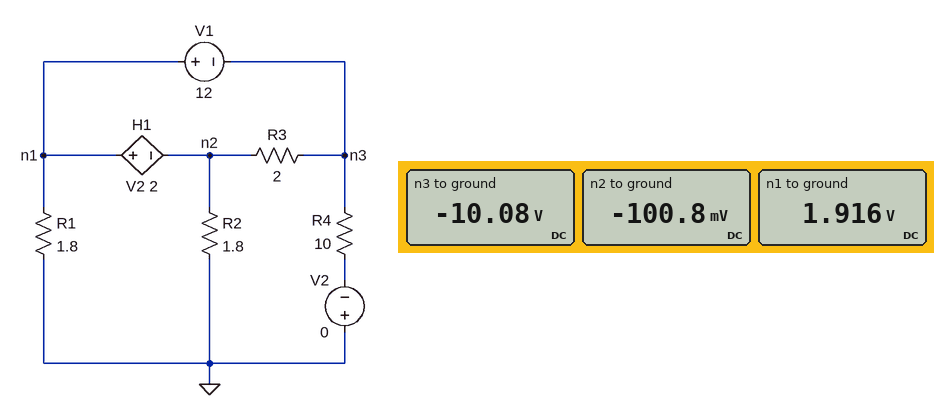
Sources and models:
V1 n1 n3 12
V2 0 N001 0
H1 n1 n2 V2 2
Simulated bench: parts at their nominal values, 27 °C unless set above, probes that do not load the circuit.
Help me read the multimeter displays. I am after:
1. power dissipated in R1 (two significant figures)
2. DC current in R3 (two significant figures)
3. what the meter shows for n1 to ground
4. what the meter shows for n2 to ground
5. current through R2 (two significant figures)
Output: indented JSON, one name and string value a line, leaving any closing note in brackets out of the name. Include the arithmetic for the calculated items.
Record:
{
  "power dissipated in R1": "(1.916 V)^2 / 1.8 Ω = 2.0 W",
  "DC current in R3": "(-100.8 mV - (-10.08 V)) / 2 Ω = 5.0 A",
  "what the meter shows for n1 to ground": "1.916 V",
  "what the meter shows for n2 to ground": "-100.8 mV",
  "current through R2": "(0 V - (-100.8 mV)) / 1.8 Ω = 56 mA"
}
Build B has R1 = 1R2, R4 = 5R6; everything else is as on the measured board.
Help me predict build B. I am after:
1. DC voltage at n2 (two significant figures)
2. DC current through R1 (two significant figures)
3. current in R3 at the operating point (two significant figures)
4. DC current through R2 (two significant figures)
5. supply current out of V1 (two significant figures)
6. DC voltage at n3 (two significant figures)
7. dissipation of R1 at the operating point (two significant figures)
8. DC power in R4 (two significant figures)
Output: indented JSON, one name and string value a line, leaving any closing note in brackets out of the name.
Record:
{
  "DC voltage at n2": "-810 mV",
  "DC current through R1": "2.1 A",
  "current in R3 at the operating point": "4.3 A",
  "DC current through R2": "450 mA",
  "supply current out of V1": "6.0 A",
  "DC voltage at n3": "-9.4 V",
  "dissipation of R1 at the operating point": "5.5 W",
  "DC power in R4": "16 W"
}
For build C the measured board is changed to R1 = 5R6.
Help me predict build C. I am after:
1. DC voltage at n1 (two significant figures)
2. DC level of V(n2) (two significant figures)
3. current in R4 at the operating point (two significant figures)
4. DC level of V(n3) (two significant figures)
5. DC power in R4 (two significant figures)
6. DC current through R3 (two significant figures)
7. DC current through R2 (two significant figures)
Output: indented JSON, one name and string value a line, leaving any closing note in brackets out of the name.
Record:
{
  "DC voltage at n1": "2.7 V",
  "DC level of V(n2)": "820 mV",
  "current in R4 at the operating point": "930 mA",
  "DC level of V(n3)": "-9.3 V",
  "DC power in R4": "8.7 W",
  "DC current through R3": "5.1 A",
  "DC current through R2": "450 mA"
}
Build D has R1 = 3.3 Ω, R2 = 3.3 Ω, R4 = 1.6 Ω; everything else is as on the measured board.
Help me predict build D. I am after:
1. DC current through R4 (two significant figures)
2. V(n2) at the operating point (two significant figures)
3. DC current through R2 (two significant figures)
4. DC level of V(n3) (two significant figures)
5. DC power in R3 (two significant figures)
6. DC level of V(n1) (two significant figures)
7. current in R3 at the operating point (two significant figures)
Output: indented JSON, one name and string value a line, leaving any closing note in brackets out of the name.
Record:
{
  "DC current through R4": "2.8 A",
  "V(n2) at the operating point": "1.8 V",
  "DC current through R2": "560 mA",
  "DC level of V(n3)": "-4.5 V",
  "DC power in R3": "20 W",
  "DC level of V(n1)": "7.5 V",
  "current in R3 at the operating point": "3.2 A"
}
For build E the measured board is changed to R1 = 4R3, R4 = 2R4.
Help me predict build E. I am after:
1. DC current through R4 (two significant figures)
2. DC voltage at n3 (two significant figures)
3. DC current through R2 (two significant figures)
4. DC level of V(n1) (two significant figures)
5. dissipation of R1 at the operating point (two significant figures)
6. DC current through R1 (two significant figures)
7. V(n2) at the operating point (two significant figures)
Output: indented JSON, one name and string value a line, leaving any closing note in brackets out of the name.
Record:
{
  "DC current through R4": "2.4 A",
  "DC voltage at n3": "-5.7 V",
  "DC current through R2": "890 mA",
  "DC level of V(n1)": "6.3 V",
  "dissipation of R1 at the operating point": "9.3 W",
  "DC current through R1": "1.5 A",
  "V(n2) at the operating point": "1.6 V"
}
